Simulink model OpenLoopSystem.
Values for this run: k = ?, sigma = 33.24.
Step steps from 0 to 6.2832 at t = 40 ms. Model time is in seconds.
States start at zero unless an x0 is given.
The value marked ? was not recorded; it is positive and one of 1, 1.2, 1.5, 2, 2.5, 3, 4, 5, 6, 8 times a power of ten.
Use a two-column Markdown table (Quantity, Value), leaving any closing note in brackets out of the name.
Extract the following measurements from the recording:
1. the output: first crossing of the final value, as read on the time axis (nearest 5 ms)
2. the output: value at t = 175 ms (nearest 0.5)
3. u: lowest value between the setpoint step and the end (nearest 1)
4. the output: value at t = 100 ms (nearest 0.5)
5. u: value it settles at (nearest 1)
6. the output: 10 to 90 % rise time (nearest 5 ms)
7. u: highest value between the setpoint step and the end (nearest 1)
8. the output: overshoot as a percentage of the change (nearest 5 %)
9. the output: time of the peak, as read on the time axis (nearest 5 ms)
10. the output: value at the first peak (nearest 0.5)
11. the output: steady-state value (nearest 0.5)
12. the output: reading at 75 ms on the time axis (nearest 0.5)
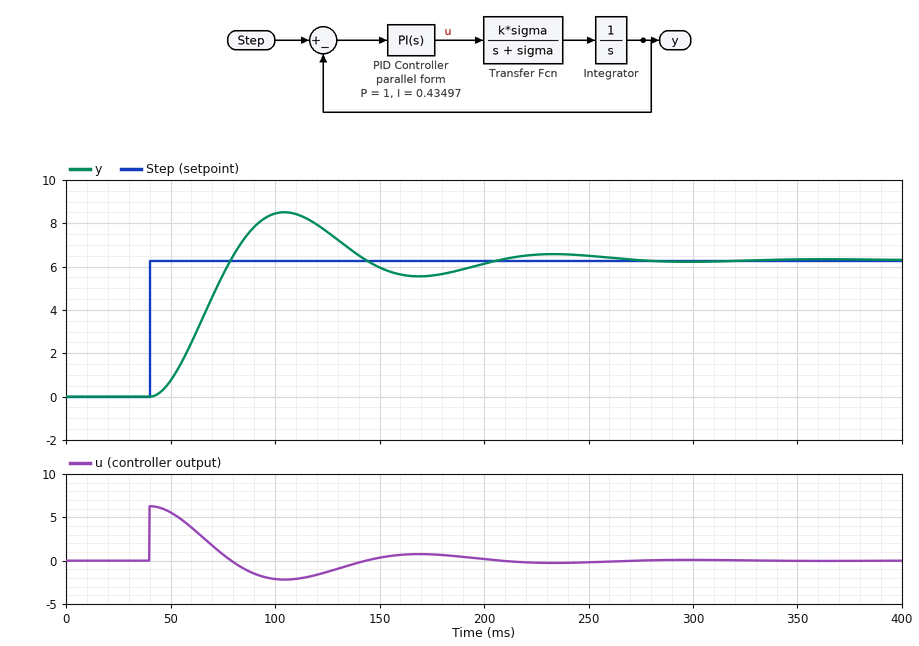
| Quantity | Value |
|---|---|
| the output: first crossing of the final value, as read on the time axis | 80 ms |
| the output: value at t = 175 ms | 5.5 |
| u: lowest value between the setpoint step and the end | -2 |
| the output: value at t = 100 ms | 8.5 |
| u: value it settles at | 0 |
| the output: 10 to 90 % rise time | 25 ms |
| u: highest value between the setpoint step and the end | 6 |
| the output: overshoot as a percentage of the change | 35 % |
| the output: time of the peak, as read on the time axis | 105 ms |
| the output: value at the first peak | 8.5 |
| the output: steady-state value | 6.5 |
| the output: reading at 75 ms on the time axis | 5.5 |
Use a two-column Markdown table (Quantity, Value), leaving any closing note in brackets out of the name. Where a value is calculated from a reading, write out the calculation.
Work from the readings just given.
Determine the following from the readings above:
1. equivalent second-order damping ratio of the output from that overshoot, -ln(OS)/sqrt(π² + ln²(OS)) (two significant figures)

| Quantity | Value |
|---|---|
| equivalent second-order damping ratio of the output from that overshoot, -ln(OS)/sqrt(π² + ln²(OS)) | ln(0.35) = -1.050; 1.050 / sqrt(9.870 + 1.102) = 0.32 |
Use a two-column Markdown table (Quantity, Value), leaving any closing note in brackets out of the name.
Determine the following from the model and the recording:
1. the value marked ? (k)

| Quantity | Value |
|---|---|
| the value marked ? | 80 |
